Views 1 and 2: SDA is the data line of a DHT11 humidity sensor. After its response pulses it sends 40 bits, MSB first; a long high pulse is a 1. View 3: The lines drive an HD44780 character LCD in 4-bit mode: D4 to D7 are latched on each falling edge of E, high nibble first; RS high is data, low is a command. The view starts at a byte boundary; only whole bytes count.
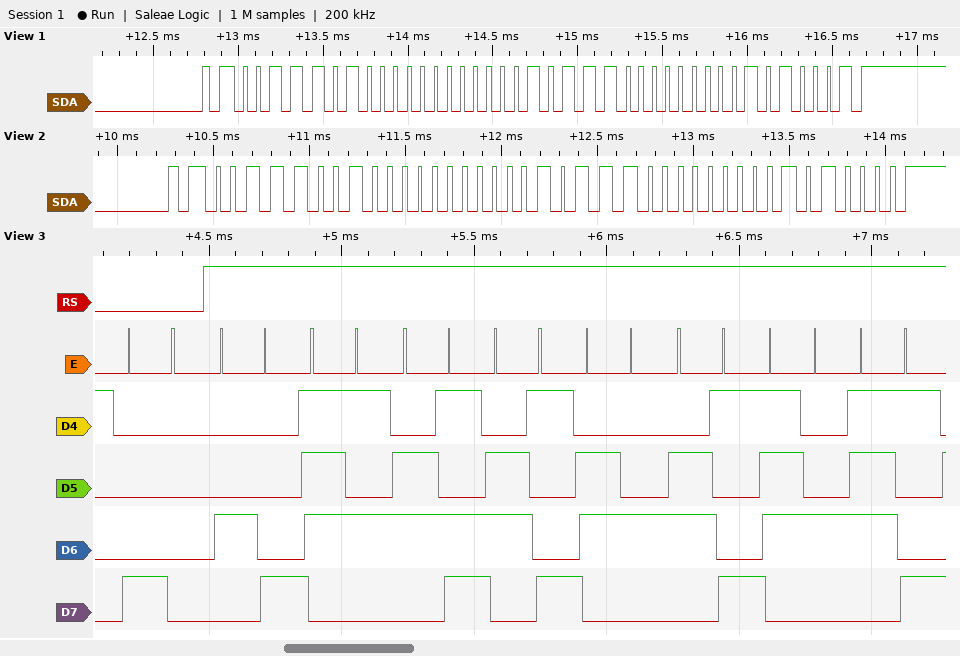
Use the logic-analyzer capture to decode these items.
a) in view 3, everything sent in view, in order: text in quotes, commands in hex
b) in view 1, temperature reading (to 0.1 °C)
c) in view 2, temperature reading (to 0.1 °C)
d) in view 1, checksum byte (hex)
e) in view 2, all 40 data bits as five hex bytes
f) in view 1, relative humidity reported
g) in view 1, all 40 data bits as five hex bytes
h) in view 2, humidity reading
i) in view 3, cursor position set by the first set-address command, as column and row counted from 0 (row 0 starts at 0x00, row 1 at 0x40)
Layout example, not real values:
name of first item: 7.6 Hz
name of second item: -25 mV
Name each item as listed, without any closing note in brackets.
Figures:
in view 3, everything sent in view, in order: text in quotes, commands in hex: 0x80 "Humidity"
in view 1, temperature reading: 23.0 °C
in view 2, temperature reading: 23.0 °C
in view 1, checksum byte: 0x51
in view 2, all 40 data bits as five hex bytes: 39 00 17 00 50
in view 1, relative humidity reported: 58 %
in view 1, all 40 data bits as five hex bytes: 3A 00 17 00 51
in view 2, humidity reading: 57 %
in view 3, cursor position set by the first set-address command, as column and row counted from 0: column 0, row 0
